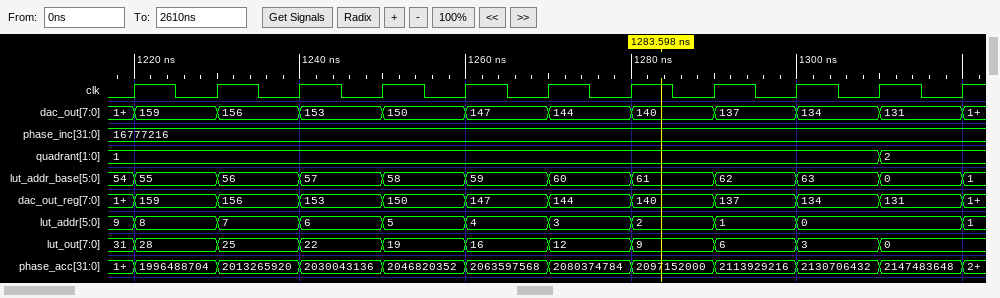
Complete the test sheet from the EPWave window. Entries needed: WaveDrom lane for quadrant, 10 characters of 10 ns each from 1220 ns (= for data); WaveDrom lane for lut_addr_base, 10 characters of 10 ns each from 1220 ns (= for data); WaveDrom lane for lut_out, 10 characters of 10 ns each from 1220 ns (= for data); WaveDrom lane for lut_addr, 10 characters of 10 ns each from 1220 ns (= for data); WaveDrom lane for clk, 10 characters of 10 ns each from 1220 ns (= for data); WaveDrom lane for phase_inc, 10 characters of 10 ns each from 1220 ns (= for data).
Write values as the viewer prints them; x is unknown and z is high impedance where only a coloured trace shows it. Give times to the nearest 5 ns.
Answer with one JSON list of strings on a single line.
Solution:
["{name: 'quadrant', wave: '=........=', data: '1 2'}", "{name: 'lut_addr_base', wave: '==========', data: '55 56 57 58 59 60 61 62 63 0'}", "{name: 'lut_out', wave: '==========', data: '28 25 22 19 16 12 9 6 3 0'}", "{name: 'lut_addr', wave: '=========.', data: '8 7 6 5 4 3 2 1 0'}", "{name: 'clk', wave: 'p.........'}", "{name: 'phase_inc', wave: '=.........', data: '16777216'}"]
